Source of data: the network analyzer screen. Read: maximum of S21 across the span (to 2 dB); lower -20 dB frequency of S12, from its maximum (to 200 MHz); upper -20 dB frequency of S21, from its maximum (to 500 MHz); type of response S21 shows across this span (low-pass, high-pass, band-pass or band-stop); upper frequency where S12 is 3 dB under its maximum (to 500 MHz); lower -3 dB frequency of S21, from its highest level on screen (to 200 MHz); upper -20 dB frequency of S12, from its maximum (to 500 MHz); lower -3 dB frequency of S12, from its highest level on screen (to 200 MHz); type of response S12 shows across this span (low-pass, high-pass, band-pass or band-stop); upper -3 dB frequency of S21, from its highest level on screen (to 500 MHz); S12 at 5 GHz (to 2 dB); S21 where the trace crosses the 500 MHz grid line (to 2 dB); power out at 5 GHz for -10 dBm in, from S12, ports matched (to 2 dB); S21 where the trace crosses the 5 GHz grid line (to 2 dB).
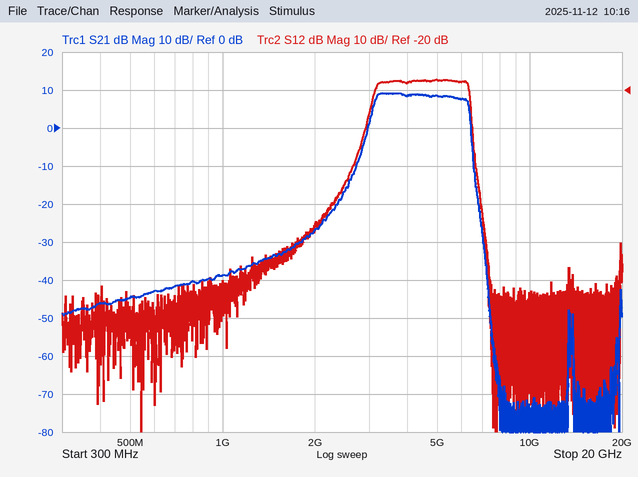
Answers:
10 dB
2.8 GHz
6.5 GHz
band-pass
6.5 GHz
3.2 GHz
6.5 GHz
3.2 GHz
band-pass
6.5 GHz
-18 dB
-44 dB
-28 dBm
8 dB
